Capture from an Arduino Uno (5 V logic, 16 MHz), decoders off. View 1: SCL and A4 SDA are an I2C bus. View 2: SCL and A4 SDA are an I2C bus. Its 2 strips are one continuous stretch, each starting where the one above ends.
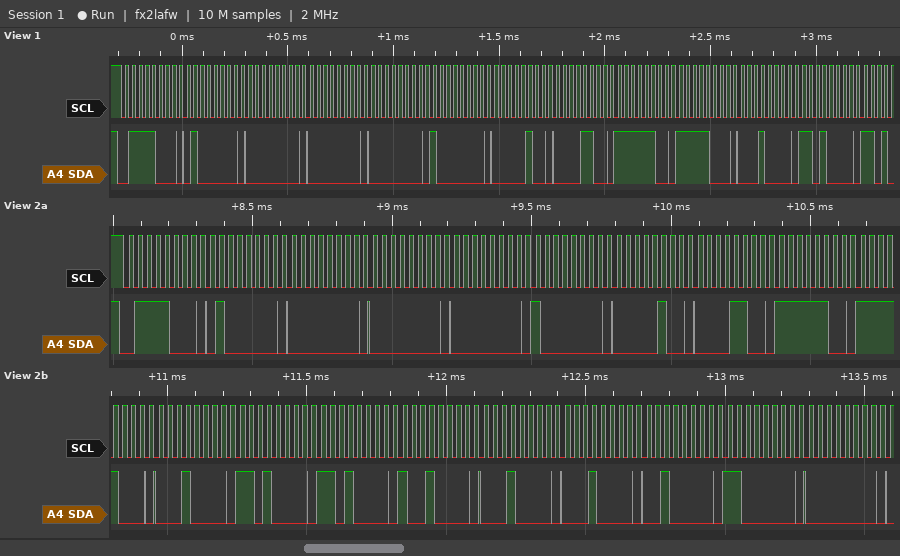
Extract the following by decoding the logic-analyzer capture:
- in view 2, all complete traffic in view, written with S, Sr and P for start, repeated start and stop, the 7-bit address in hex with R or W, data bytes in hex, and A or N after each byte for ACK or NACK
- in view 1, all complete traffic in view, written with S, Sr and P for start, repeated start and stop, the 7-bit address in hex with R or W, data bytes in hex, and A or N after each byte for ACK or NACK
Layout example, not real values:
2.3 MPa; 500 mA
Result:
S 3CW A 40 A 00 A 00 A 00 A 80 A 04 A 0C A FC A F8 A 10 A D0 A D0 A 90 A 10 A 10 A 20 A C0 A 00 A; S 3CW A 40 A 00 A 00 A 00 A 80 A 04 A 0C A FC A F8 A 10 A D0 A
